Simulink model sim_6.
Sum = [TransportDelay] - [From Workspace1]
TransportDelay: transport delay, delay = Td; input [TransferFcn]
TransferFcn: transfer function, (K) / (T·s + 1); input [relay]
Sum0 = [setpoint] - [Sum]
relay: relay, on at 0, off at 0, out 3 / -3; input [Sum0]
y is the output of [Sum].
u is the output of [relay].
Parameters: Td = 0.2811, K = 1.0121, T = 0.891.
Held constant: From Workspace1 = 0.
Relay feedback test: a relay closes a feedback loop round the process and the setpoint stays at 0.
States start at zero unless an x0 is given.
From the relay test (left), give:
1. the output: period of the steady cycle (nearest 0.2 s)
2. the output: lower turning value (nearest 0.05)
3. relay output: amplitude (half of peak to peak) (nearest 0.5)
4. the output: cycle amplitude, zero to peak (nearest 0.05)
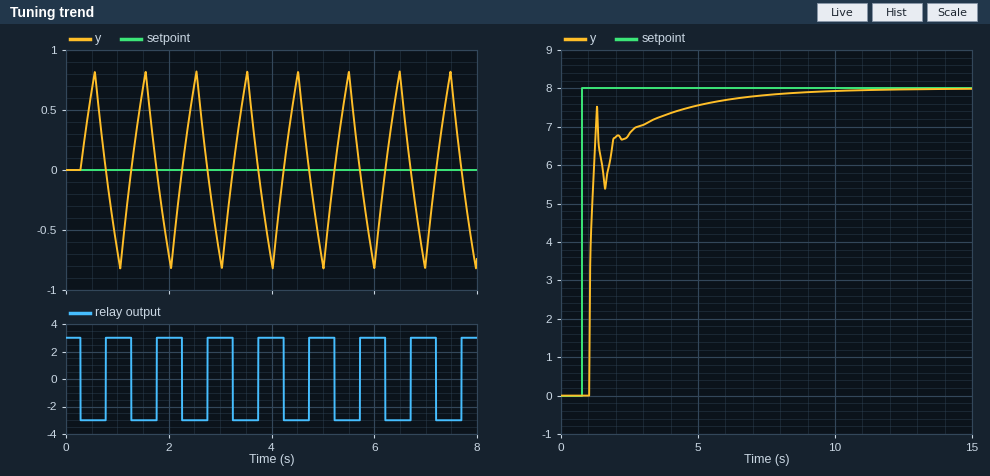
1.0 s
-0.80
3.0
0.80
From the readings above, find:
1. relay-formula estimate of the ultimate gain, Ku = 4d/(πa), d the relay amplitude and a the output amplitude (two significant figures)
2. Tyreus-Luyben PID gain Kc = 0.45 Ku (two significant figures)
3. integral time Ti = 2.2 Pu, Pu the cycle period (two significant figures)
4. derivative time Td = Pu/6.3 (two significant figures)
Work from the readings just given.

4.8
2.2
2.2 s
0.16 s
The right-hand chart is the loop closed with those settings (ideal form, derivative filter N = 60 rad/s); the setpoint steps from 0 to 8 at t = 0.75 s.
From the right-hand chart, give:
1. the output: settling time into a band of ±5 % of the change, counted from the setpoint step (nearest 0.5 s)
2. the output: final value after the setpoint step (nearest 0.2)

4.5 s
8.0
